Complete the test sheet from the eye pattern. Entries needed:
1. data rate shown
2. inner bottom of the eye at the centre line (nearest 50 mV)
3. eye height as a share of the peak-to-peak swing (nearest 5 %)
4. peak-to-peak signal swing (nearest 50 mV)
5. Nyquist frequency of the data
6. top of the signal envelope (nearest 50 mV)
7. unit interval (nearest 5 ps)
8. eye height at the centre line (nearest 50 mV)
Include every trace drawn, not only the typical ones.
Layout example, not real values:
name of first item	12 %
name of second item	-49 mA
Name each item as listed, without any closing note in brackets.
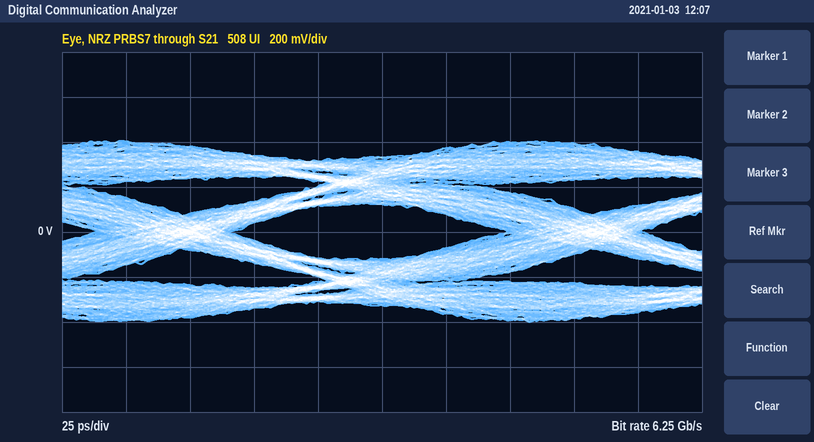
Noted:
data rate shown	6.25 Gb/s
inner bottom of the eye at the centre line	-100 mV
eye height as a share of the peak-to-peak swing	30 %
peak-to-peak signal swing	800 mV
Nyquist frequency of the data	3.125 GHz
top of the signal envelope	400 mV
unit interval	160 ps
eye height at the centre line	250 mV
